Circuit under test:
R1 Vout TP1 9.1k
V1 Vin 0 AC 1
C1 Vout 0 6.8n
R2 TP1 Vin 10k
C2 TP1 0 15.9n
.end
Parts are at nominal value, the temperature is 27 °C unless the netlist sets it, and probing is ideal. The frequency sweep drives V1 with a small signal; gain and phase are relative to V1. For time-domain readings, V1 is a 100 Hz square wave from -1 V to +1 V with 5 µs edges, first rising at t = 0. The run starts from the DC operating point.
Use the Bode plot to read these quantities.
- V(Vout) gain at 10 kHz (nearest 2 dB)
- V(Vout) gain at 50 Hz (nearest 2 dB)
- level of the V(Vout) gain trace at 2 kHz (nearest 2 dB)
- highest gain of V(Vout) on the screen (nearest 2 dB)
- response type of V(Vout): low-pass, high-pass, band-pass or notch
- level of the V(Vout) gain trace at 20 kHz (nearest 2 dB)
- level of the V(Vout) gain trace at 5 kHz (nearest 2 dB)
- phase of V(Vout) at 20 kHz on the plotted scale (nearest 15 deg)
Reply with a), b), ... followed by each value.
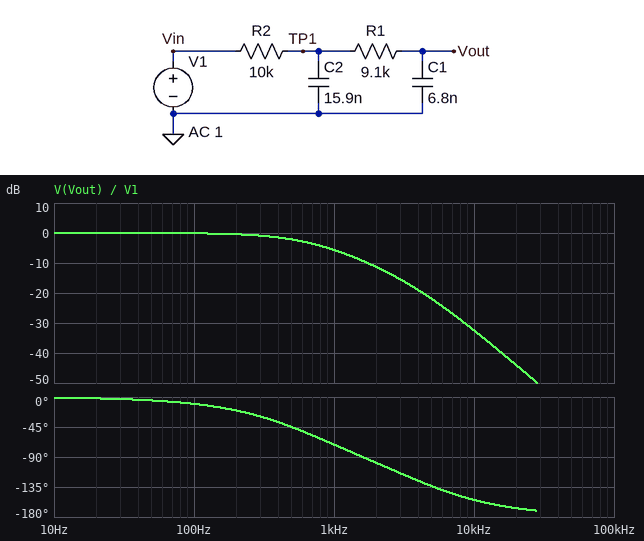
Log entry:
a) -32 dB
b) 0 dB
c) -12 dB
d) 0 dB
e) low-pass
f) -44 dB
g) -22 dB
h) -165 deg
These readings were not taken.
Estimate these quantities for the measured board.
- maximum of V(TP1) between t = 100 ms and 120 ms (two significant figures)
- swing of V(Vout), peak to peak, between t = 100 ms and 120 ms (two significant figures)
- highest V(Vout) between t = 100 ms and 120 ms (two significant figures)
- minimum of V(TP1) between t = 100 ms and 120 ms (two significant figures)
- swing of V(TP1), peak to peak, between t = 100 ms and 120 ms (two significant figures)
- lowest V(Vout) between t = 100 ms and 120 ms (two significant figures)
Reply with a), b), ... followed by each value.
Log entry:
a) 1.0 V
b) 2.0 V
c) 1.0 V
d) -1.0 V
e) 2.0 V
f) -1.0 V
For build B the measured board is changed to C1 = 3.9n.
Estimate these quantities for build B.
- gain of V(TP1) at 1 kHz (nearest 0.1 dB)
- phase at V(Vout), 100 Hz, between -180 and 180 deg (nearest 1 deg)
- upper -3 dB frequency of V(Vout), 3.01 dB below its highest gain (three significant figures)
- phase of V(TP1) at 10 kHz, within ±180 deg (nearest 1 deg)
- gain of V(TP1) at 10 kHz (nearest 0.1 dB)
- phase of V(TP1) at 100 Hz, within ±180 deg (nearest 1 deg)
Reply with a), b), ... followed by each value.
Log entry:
a) -4.2 dB
b) -8 deg
c) 759 Hz
d) -80 deg
e) -20.5 dB
f) -7 deg
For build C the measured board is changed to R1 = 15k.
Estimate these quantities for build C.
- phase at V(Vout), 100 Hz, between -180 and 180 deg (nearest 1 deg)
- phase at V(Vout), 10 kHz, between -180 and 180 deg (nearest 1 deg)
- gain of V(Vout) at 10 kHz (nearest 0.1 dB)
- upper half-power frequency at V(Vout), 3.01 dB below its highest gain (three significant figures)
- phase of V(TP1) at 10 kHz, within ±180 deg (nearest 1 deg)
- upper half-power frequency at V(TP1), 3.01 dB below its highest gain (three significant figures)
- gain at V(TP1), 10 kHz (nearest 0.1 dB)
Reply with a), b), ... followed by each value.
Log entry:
a) -12 deg
b) -162 deg
c) -36.4 dB
d) 566 Hz
e) -81 deg
f) 653 Hz
g) -20.2 dB
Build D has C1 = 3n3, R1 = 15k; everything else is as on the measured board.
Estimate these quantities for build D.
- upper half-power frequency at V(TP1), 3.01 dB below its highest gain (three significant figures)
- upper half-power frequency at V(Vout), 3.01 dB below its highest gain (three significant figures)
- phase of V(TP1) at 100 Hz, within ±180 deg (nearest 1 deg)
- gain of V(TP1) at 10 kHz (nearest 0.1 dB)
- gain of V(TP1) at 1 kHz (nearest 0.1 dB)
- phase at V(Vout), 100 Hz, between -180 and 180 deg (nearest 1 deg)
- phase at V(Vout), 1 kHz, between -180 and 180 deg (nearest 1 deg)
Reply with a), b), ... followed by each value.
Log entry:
a) 803 Hz
b) 759 Hz
c) -7 deg
d) -20.3 dB
e) -4.0 dB
f) -9 deg
g) -66 deg
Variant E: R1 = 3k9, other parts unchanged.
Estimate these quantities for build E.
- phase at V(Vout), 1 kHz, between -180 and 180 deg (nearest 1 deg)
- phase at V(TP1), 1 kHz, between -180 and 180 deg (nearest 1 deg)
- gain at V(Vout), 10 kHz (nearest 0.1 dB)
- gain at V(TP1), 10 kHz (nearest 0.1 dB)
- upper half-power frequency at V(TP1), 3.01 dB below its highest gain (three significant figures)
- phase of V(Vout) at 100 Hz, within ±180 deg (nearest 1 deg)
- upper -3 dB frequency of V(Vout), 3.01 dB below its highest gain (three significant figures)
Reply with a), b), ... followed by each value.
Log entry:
a) -62 deg
b) -53 deg
c) -27.0 dB
d) -21.2 dB
e) 680 Hz
f) -9 deg
g) 672 Hz
